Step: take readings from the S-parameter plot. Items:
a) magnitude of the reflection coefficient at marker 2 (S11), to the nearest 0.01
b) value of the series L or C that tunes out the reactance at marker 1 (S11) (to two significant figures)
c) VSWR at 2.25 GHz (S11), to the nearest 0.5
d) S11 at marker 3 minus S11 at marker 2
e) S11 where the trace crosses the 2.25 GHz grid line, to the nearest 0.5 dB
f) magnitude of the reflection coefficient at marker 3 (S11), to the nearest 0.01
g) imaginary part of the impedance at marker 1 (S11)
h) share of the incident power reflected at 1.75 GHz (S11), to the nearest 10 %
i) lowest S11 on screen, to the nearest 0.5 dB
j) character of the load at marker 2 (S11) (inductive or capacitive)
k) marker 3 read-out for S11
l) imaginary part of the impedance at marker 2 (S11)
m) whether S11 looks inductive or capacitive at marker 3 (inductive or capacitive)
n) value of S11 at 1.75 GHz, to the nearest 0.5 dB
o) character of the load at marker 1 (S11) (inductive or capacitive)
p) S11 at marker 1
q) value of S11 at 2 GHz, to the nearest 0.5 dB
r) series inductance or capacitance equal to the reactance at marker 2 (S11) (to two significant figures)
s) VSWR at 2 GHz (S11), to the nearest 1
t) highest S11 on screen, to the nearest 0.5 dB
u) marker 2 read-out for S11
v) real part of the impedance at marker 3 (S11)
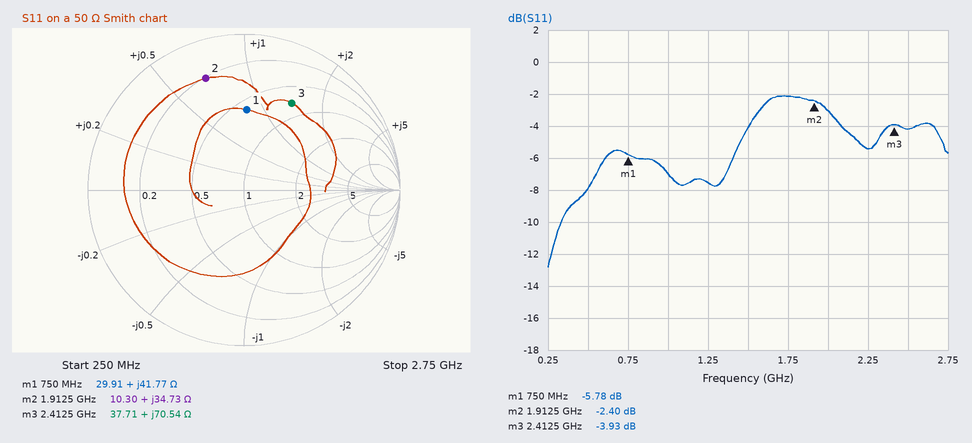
0.76
5.1 pF
3.5
-1.53 dB
-5.5 dB
0.64
+41.77 Ω
60 %
-13.0 dB
inductive
-3.93 dB
+34.73 Ω
inductive
-2.0 dB
inductive
-5.78 dB
-3.0 dB
2.9 nH
6
-2.0 dB
-2.40 dB
37.71 Ω
